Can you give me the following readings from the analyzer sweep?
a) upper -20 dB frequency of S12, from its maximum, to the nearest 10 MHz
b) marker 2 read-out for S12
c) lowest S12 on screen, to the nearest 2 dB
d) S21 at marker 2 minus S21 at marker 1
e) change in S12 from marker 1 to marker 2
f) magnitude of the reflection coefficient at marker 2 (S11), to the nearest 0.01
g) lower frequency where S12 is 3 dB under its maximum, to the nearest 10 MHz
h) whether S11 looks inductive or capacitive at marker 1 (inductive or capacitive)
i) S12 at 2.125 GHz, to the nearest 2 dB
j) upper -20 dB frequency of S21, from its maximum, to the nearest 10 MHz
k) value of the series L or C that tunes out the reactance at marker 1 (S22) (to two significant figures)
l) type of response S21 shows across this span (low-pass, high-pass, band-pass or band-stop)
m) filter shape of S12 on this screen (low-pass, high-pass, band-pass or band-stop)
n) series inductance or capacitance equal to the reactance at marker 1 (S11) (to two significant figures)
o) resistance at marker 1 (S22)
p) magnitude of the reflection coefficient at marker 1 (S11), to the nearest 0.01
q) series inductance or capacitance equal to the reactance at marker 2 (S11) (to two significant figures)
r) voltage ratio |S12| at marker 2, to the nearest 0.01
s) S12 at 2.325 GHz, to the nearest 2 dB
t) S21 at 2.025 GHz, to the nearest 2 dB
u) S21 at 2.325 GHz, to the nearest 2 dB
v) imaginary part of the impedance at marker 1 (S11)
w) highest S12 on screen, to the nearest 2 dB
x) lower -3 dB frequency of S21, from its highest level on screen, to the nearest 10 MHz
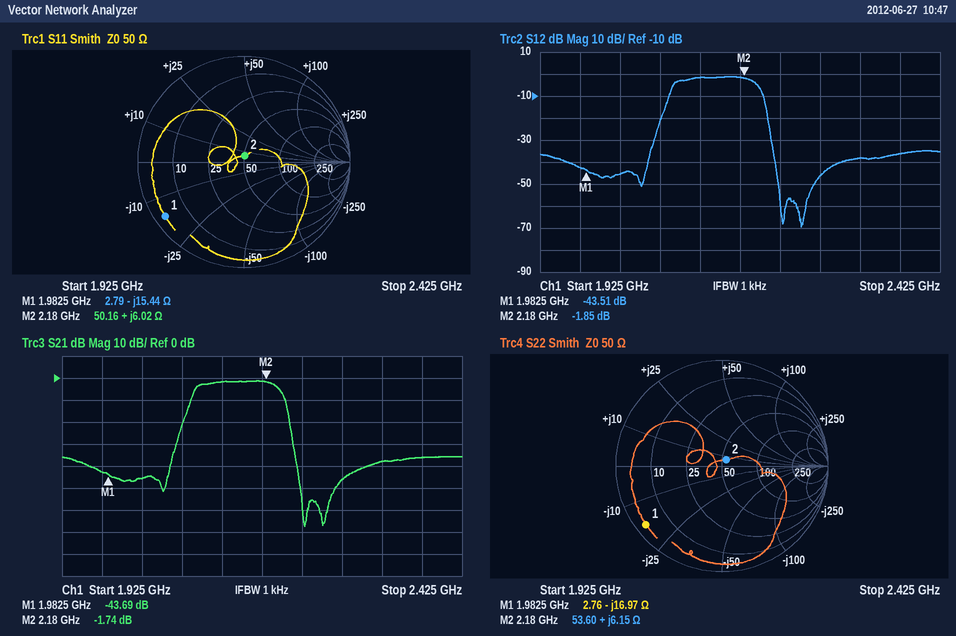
2.21 GHz
-1.85 dB
-70 dB
41.95 dB
41.66 dB
0.06
2.09 GHz
capacitive
-2 dB
2.21 GHz
1.4 nH
band-pass
band-pass
5.2 pF
2.76 Ω
0.90
440 pH
0.81
-38 dB
-46 dB
-38 dB
-15.44 Ω
-2 dB
2.09 GHz
